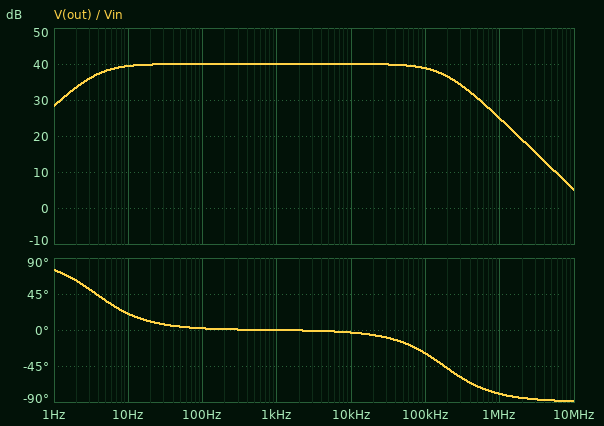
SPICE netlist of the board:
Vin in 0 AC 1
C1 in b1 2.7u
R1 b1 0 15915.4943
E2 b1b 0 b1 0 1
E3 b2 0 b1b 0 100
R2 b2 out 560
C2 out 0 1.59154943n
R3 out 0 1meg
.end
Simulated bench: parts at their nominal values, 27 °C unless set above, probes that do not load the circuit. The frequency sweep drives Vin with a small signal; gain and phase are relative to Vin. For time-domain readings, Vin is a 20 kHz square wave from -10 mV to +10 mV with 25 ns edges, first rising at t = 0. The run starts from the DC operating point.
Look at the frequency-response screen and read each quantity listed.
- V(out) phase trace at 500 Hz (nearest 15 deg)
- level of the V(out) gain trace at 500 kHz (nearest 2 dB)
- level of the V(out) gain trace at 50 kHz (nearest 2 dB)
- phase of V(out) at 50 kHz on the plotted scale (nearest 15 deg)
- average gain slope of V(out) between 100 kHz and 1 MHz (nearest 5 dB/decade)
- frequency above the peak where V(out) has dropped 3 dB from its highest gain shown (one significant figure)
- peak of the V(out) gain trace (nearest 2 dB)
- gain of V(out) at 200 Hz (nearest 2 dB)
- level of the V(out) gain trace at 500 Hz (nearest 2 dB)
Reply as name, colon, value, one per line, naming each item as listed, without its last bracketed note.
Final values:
V(out) phase trace at 500 Hz: 0 deg
level of the V(out) gain trace at 500 kHz: 30 dB
level of the V(out) gain trace at 50 kHz: 40 dB
phase of V(out) at 50 kHz on the plotted scale: -15 deg
average gain slope of V(out) between 100 kHz and 1 MHz: -15 dB/decade
frequency above the peak where V(out) has dropped 3 dB from its highest gain shown: 200 kHz
peak of the V(out) gain trace: 40 dB
gain of V(out) at 200 Hz: 40 dB
level of the V(out) gain trace at 500 Hz: 40 dB
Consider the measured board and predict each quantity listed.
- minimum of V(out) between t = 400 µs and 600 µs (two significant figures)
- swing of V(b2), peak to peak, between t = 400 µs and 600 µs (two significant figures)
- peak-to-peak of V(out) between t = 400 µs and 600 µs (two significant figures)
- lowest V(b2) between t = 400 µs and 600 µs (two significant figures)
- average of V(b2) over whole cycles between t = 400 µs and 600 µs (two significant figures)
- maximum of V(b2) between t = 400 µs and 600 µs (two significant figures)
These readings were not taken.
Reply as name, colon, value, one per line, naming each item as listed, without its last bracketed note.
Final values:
minimum of V(out) between t = 400 µs and 600 µs: -14 mV
swing of V(b2), peak to peak, between t = 400 µs and 600 µs: 2.0 V
peak-to-peak of V(out) between t = 400 µs and 600 µs: 2.0 V
lowest V(b2) between t = 400 µs and 600 µs: -14 mV
average of V(b2) over whole cycles between t = 400 µs and 600 µs: 990 mV
maximum of V(b2) between t = 400 µs and 600 µs: 2.0 V
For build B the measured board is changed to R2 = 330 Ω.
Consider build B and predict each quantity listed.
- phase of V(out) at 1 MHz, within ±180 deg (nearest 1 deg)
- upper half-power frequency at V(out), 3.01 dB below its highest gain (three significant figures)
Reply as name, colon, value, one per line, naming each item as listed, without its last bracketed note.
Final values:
phase of V(out) at 1 MHz, within ±180 deg: -73 deg
upper half-power frequency at V(out), 3.01 dB below its highest gain: 303 kHz
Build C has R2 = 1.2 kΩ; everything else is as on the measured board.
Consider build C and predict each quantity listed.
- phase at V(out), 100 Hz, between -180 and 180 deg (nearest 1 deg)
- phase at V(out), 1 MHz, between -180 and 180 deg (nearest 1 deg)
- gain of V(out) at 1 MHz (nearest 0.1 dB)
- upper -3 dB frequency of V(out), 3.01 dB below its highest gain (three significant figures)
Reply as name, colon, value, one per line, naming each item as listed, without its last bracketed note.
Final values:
phase at V(out), 100 Hz, between -180 and 180 deg: 2 deg
phase at V(out), 1 MHz, between -180 and 180 deg: -85 deg
gain of V(out) at 1 MHz: 18.4 dB
upper -3 dB frequency of V(out), 3.01 dB below its highest gain: 83.4 kHz
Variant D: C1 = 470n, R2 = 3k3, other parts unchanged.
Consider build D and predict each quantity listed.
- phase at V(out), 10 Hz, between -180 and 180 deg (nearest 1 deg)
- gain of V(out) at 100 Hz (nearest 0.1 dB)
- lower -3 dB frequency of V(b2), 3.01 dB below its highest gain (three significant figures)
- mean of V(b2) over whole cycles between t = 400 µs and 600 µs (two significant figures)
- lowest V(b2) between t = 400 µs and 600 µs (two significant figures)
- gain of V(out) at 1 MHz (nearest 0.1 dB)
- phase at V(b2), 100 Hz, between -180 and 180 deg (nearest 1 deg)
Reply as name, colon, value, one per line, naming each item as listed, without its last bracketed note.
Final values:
phase at V(out), 10 Hz, between -180 and 180 deg: 65 deg
gain of V(out) at 100 Hz: 39.8 dB
lower -3 dB frequency of V(b2), 3.01 dB below its highest gain: 21.3 Hz
mean of V(b2) over whole cycles between t = 400 µs and 600 µs: 930 mV
lowest V(b2) between t = 400 µs and 600 µs: -77 mV
gain of V(out) at 1 MHz: 9.6 dB
phase at V(b2), 100 Hz, between -180 and 180 deg: 12 deg
